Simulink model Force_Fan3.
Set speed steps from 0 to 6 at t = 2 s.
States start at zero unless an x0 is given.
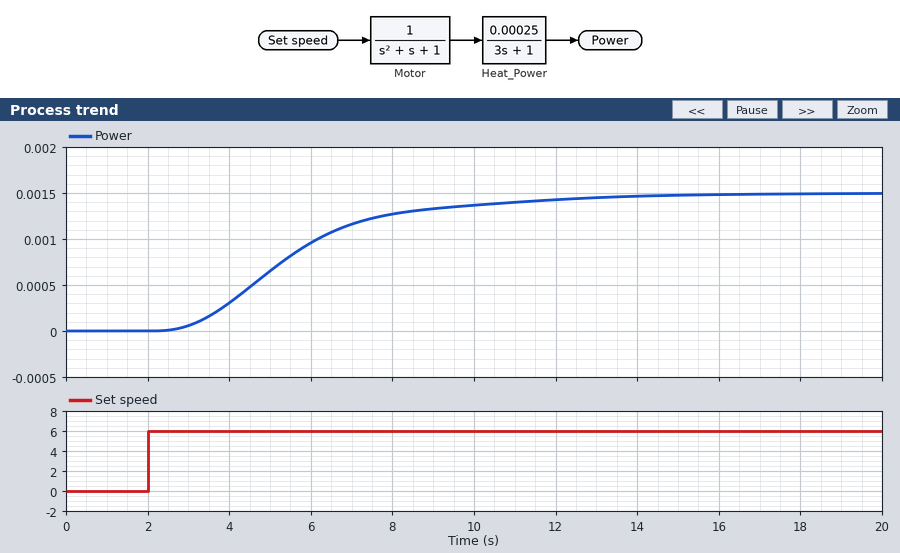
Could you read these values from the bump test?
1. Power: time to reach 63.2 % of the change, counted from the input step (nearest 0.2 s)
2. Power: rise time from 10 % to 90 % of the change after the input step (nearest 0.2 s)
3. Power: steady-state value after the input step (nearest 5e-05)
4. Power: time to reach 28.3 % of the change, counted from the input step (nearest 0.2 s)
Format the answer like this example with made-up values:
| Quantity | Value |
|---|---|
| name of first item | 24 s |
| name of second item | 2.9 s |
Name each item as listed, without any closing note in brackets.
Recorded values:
| Quantity | Value |
|---|---|
| Power: time to reach 63.2 % of the change, counted from the input step | 4.0 s |
| Power: rise time from 10 % to 90 % of the change after the input step | 6.0 s |
| Power: steady-state value after the input step | 0.00150 |
| Power: time to reach 28.3 % of the change, counted from the input step | 2.4 s |
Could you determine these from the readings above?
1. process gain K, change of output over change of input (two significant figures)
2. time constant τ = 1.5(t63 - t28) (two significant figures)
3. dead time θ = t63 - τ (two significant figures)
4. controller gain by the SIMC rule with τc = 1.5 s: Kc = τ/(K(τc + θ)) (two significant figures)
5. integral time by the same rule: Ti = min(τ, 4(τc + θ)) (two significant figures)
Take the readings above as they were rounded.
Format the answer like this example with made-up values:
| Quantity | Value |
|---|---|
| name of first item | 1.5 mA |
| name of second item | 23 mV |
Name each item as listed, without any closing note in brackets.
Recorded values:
| Quantity | Value |
|---|---|
| process gain K, change of output over change of input | 0.00025 |
| time constant τ = 1.5(t63 - t28) | 2.4 s |
| dead time θ = t63 - τ | 1.6 s |
| controller gain by the SIMC rule with τc = 1.5 s: Kc = τ/(K(τc + θ)) | 3100 |
| integral time by the same rule: Ti = min(τ, 4(τc + θ)) | 2.4 s |
